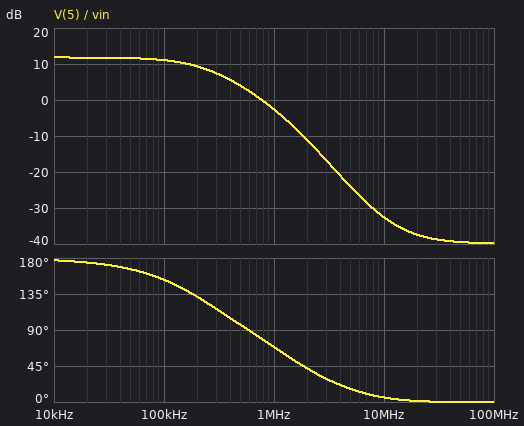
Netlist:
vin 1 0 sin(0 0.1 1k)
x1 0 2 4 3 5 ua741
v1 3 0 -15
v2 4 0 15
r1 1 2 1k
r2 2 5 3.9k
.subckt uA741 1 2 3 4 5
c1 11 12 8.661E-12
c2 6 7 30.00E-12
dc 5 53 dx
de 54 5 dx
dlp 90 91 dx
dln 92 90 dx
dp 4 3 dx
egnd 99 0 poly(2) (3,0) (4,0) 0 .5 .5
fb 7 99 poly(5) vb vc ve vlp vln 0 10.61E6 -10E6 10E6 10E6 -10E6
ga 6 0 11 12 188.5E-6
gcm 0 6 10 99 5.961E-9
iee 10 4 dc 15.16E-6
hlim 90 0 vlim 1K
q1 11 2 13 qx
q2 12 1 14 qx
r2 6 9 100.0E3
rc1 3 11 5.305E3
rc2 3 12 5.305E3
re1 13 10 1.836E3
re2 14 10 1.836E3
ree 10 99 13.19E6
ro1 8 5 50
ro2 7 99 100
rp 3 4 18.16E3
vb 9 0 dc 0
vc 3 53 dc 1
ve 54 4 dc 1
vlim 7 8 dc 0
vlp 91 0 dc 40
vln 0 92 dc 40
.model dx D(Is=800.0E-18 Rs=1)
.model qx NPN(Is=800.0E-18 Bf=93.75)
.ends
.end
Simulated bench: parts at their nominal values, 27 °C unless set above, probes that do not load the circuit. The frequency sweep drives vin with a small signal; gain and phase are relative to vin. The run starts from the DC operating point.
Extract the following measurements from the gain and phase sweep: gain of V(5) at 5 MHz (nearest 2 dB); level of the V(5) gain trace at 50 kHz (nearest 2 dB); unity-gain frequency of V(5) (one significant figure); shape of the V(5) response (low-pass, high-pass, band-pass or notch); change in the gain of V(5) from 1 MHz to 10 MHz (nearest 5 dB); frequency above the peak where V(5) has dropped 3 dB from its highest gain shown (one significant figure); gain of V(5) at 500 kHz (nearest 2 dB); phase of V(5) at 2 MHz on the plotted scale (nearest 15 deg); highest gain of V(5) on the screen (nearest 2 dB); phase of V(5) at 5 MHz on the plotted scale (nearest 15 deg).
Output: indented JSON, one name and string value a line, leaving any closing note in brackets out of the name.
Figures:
{
  "gain of V(5) at 5 MHz": "-24 dB",
  "level of the V(5) gain trace at 50 kHz": "12 dB",
  "unity-gain frequency of V(5)": "800 kHz",
  "shape of the V(5) response": "low-pass",
  "change in the gain of V(5) from 1 MHz to 10 MHz": "-30 dB",
  "frequency above the peak where V(5) has dropped 3 dB from its highest gain shown": "200 kHz",
  "gain of V(5) at 500 kHz": "4 dB",
  "phase of V(5) at 2 MHz on the plotted scale": "45 deg",
  "highest gain of V(5) on the screen": "12 dB",
  "phase of V(5) at 5 MHz on the plotted scale": "15 deg"
}
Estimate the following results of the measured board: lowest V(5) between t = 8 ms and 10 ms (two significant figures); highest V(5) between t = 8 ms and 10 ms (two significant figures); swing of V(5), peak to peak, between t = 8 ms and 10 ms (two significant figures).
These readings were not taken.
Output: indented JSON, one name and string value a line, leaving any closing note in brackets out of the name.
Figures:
{
  "lowest V(5) between t = 8 ms and 10 ms": "-390 mV",
  "highest V(5) between t = 8 ms and 10 ms": "390 mV",
  "swing of V(5), peak to peak, between t = 8 ms and 10 ms": "780 mV"
}
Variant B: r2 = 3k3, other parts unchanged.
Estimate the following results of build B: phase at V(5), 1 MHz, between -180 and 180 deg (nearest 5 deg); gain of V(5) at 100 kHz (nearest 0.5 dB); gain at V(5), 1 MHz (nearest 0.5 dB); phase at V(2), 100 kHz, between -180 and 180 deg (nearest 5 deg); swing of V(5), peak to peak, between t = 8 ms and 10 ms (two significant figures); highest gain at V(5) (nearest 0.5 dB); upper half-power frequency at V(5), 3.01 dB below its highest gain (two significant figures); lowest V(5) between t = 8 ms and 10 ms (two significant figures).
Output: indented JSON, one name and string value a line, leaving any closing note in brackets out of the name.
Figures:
{
  "phase at V(5), 1 MHz, between -180 and 180 deg": "70 deg",
  "gain of V(5) at 100 kHz": "10.0 dB",
  "gain at V(5), 1 MHz": "-3.0 dB",
  "phase at V(2), 100 kHz, between -180 and 180 deg": "70 deg",
  "swing of V(5), peak to peak, between t = 8 ms and 10 ms": "660 mV",
  "highest gain at V(5)": "10.5 dB",
  "upper half-power frequency at V(5), 3.01 dB below its highest gain": "260 kHz",
  "lowest V(5) between t = 8 ms and 10 ms": "-330 mV"
}
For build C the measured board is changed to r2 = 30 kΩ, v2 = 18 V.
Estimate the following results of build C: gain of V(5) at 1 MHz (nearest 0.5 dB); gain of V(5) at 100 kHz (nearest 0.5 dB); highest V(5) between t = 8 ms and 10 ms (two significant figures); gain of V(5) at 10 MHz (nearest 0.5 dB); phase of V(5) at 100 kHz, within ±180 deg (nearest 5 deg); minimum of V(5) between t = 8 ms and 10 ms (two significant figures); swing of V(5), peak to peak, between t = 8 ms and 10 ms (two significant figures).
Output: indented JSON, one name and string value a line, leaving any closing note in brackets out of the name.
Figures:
{
  "gain of V(5) at 1 MHz": "-1.5 dB",
  "gain of V(5) at 100 kHz": "19.5 dB",
  "highest V(5) between t = 8 ms and 10 ms": "3.0 V",
  "gain of V(5) at 10 MHz": "-35.0 dB",
  "phase of V(5) at 100 kHz, within ±180 deg": "105 deg",
  "minimum of V(5) between t = 8 ms and 10 ms": "-3.0 V",
  "swing of V(5), peak to peak, between t = 8 ms and 10 ms": "6.0 V"
}
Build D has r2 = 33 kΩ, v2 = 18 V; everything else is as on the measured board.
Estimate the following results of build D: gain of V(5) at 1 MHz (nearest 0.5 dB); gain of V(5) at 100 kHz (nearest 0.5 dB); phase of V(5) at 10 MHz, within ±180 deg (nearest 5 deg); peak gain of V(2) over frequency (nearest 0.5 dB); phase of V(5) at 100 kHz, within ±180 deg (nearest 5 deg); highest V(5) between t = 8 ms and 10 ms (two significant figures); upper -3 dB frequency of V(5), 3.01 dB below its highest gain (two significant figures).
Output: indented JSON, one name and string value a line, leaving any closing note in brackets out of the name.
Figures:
{
  "gain of V(5) at 1 MHz": "-1.5 dB",
  "gain of V(5) at 100 kHz": "19.5 dB",
  "phase of V(5) at 10 MHz, within ±180 deg": "10 deg",
  "peak gain of V(2) over frequency": "0 dB",
  "phase of V(5) at 100 kHz, within ±180 deg": "105 deg",
  "highest V(5) between t = 8 ms and 10 ms": "3.3 V",
  "upper -3 dB frequency of V(5), 3.01 dB below its highest gain": "30 kHz"
}
